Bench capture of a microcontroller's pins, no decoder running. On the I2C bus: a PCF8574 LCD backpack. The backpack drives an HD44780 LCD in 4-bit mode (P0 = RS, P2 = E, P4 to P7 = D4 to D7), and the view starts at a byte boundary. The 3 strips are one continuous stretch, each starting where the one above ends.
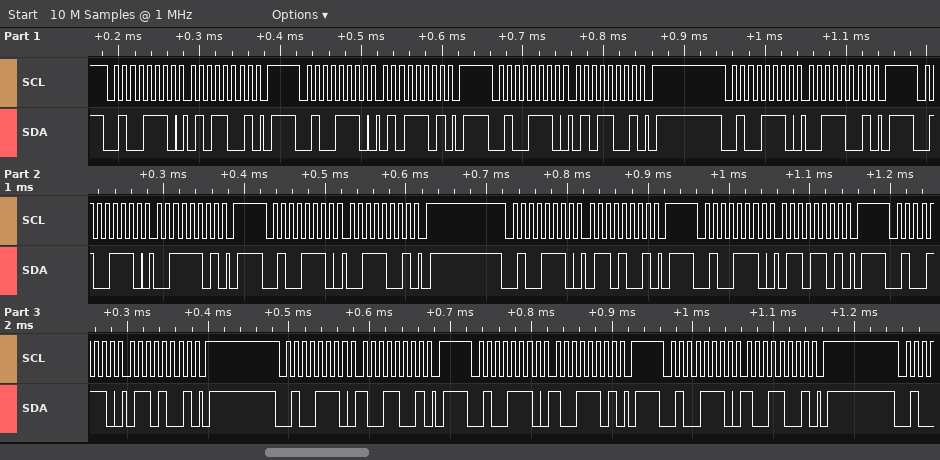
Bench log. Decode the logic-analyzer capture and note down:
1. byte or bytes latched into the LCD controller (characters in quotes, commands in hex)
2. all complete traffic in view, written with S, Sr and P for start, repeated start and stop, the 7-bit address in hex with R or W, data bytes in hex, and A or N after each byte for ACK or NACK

'S' 'i'
S 27W A 59 A P S 27W A 5D A P S 27W A 59 A P S 27W A 39 A P S 27W A 3D A P S 27W A 39 A P S 27W A 69 A P S 27W A 6D A P S 27W A 69 A P S 27W A 99 A P S 27W A 9D A P S 27W A 99 A P
